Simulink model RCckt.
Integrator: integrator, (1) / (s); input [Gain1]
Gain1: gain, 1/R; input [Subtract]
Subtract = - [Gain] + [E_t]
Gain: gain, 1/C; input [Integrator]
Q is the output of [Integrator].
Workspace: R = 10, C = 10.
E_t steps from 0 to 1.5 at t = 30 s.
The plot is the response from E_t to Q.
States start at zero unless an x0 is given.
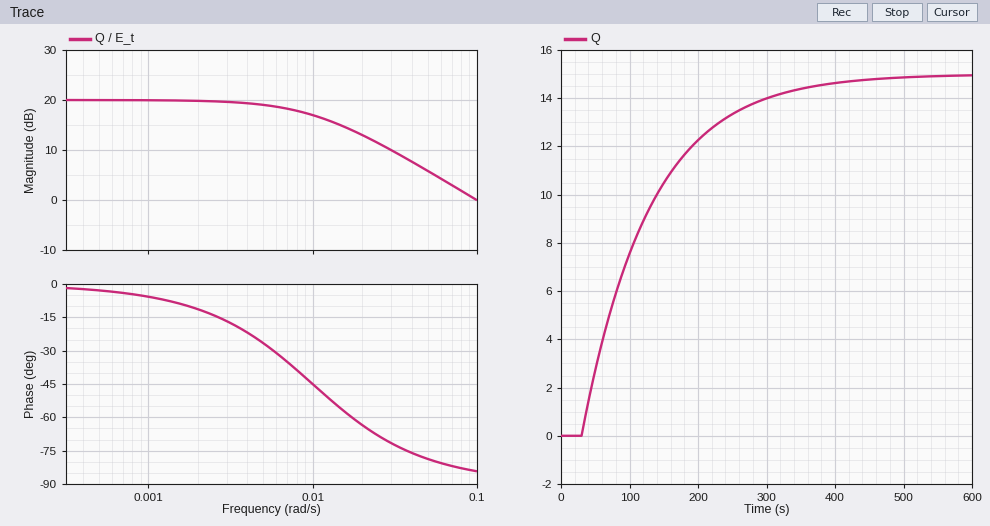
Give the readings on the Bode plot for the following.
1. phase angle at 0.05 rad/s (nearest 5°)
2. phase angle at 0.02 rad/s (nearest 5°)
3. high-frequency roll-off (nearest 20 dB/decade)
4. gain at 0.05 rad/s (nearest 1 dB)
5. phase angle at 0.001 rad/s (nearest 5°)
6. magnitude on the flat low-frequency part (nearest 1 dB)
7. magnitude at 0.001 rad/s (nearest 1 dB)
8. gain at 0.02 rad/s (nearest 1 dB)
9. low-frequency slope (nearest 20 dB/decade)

-80°
-65°
-20 dB/decade
6 dB
-5°
20 dB
20 dB
13 dB
0 dB/decade
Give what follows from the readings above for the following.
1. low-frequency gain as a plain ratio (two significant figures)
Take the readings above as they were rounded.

10
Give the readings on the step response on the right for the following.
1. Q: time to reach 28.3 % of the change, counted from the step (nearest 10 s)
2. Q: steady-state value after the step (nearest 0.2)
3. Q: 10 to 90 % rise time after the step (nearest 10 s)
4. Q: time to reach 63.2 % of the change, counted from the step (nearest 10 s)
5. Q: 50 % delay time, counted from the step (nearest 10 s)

30 s
15.0
220 s
100 s
70 s
